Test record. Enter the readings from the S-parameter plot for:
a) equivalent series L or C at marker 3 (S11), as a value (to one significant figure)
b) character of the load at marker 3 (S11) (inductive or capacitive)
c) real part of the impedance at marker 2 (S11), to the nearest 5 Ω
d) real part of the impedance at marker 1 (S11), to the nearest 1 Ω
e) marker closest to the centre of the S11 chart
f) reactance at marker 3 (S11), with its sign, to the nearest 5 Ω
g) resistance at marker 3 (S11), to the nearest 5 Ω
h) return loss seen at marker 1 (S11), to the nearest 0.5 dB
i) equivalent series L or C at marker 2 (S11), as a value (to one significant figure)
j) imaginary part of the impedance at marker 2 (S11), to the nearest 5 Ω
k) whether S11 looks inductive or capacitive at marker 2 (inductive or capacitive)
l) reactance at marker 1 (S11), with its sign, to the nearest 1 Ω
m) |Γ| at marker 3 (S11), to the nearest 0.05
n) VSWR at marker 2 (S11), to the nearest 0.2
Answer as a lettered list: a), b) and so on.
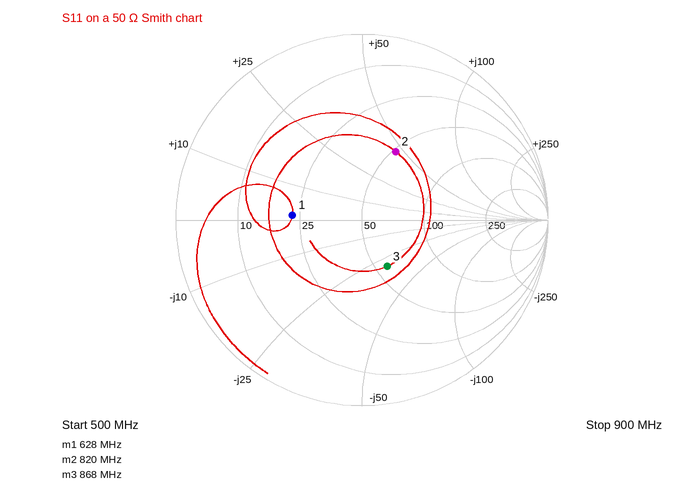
a) 6 pF
b) capacitive
c) 50 Ω
d) 23 Ω
e) marker 3
f) -30 Ω
g) 55 Ω
h) 8.5 dB
i) 9 nH
j) +45 Ω
k) inductive
l) +1 Ω
m) 0.30
n) 2.4
